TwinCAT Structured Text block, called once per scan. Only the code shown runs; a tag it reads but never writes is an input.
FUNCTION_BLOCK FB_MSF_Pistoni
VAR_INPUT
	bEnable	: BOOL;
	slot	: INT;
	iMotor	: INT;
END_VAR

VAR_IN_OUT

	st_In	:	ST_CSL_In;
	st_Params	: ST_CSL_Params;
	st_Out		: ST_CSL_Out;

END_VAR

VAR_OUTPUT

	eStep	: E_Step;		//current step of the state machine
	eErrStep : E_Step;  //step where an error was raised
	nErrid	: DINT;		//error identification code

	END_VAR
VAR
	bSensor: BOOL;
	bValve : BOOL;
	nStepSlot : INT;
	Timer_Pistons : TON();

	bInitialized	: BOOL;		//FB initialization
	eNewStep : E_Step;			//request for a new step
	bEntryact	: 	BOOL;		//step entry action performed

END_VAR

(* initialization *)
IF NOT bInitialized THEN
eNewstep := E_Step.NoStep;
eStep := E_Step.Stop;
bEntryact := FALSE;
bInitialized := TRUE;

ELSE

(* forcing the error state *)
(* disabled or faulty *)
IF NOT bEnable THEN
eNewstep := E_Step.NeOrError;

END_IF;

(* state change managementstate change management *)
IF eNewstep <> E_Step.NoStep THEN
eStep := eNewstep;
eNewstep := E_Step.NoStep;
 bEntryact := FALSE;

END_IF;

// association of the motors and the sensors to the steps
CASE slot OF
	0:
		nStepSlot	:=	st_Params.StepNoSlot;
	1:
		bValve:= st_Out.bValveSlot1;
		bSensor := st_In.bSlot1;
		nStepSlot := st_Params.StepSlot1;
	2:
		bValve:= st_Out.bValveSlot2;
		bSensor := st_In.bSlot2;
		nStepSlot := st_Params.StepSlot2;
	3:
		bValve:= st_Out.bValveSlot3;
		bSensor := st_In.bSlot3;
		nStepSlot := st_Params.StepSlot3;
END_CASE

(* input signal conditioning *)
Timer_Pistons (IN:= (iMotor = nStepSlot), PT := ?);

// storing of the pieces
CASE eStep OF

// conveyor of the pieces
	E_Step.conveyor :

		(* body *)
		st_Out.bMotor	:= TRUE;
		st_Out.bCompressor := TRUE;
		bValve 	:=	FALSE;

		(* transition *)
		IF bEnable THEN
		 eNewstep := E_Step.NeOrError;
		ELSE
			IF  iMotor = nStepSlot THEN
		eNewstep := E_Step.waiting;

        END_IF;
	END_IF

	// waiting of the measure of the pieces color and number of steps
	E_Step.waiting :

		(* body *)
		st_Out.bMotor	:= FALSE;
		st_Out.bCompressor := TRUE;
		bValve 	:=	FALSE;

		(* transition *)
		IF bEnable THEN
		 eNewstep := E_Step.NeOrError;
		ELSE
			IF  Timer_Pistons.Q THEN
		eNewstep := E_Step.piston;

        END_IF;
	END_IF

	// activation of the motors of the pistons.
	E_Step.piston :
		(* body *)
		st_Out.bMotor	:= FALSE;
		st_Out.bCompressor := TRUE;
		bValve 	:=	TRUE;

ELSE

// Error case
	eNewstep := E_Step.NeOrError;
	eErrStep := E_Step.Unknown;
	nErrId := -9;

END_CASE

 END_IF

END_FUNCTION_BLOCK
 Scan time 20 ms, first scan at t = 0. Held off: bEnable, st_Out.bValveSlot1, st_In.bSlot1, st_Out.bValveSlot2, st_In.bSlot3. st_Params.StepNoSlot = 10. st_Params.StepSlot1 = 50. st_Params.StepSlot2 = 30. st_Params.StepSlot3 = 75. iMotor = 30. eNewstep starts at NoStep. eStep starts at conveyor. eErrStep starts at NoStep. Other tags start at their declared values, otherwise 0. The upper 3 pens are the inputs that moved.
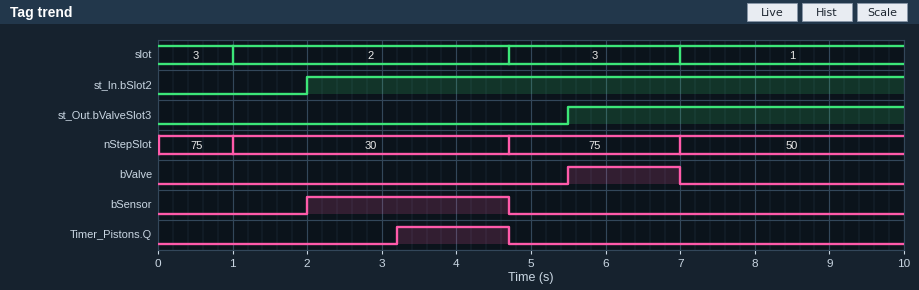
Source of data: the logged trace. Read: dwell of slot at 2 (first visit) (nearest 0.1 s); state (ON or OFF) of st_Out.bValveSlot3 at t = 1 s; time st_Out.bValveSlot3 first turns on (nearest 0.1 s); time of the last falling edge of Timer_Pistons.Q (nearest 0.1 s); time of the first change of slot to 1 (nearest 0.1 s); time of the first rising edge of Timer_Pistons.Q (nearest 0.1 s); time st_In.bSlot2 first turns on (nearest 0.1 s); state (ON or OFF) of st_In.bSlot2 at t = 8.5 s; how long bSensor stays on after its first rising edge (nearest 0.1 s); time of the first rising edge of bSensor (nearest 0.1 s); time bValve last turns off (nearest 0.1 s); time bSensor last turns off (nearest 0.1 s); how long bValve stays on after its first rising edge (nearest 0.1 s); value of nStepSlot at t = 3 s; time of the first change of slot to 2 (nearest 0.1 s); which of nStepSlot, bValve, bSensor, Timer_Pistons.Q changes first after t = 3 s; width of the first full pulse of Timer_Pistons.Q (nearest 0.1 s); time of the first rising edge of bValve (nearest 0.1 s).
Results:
3.7 s
OFF
5.5 s
4.7 s
7.0 s
3.2 s
2.0 s
ON
2.7 s
2.0 s
7.0 s
4.7 s
1.5 s
30
1.0 s
Timer_Pistons.Q
1.5 s
5.5 s
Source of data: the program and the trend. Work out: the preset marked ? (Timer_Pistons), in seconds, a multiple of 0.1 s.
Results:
2.2 s
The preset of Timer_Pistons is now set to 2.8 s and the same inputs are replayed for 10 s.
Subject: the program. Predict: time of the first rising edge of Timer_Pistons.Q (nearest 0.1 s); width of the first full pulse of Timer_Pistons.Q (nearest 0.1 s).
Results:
3.8 s
0.9 s
